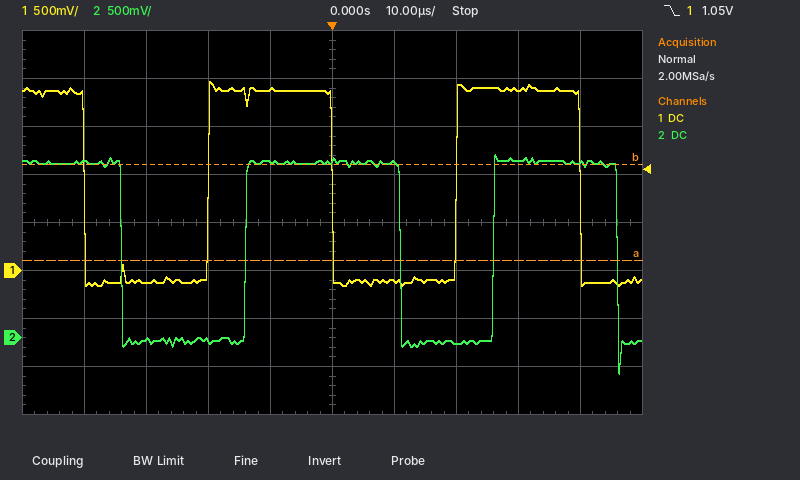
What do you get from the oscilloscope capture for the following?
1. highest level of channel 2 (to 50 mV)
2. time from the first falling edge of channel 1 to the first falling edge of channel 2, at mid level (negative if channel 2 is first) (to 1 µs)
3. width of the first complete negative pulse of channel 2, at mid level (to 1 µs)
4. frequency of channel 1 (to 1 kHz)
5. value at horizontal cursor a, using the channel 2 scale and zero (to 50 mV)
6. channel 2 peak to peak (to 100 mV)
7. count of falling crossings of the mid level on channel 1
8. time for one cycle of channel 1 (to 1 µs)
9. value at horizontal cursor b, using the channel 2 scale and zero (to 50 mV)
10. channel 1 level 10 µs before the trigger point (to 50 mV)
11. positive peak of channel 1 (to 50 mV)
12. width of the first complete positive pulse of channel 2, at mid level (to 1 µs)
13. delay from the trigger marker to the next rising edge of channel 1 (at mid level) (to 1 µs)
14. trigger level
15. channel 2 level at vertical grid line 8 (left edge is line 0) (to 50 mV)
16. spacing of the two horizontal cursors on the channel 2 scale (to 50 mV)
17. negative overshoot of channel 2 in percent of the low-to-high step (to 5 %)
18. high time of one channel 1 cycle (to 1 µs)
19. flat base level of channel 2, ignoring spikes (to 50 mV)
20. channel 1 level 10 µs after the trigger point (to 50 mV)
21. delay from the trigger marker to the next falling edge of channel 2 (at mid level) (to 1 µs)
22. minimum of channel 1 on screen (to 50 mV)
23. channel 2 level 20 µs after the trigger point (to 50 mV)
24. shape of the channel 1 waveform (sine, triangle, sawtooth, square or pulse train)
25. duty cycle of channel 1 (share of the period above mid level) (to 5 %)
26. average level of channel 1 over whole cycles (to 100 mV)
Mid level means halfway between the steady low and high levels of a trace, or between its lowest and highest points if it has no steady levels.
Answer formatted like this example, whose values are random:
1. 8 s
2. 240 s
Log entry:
1. 1.90 V
2. +6 µs
3. 20 µs
4. 25 kHz
5. 800 mV
6. 2.30 V
7. 3
8. 40 µs
9. 1.80 V
10. 1.90 V
11. 1.95 V
12. 25 µs
13. 20 µs
14. 1.05 V
15. 1.85 V
16. 1.00 V
17. 20 %
18. 20 µs
19. -50 mV
20. -100 mV
21. 11 µs
22. -150 mV
23. -50 mV
24. square
25. 50 %
26. 900 mV
